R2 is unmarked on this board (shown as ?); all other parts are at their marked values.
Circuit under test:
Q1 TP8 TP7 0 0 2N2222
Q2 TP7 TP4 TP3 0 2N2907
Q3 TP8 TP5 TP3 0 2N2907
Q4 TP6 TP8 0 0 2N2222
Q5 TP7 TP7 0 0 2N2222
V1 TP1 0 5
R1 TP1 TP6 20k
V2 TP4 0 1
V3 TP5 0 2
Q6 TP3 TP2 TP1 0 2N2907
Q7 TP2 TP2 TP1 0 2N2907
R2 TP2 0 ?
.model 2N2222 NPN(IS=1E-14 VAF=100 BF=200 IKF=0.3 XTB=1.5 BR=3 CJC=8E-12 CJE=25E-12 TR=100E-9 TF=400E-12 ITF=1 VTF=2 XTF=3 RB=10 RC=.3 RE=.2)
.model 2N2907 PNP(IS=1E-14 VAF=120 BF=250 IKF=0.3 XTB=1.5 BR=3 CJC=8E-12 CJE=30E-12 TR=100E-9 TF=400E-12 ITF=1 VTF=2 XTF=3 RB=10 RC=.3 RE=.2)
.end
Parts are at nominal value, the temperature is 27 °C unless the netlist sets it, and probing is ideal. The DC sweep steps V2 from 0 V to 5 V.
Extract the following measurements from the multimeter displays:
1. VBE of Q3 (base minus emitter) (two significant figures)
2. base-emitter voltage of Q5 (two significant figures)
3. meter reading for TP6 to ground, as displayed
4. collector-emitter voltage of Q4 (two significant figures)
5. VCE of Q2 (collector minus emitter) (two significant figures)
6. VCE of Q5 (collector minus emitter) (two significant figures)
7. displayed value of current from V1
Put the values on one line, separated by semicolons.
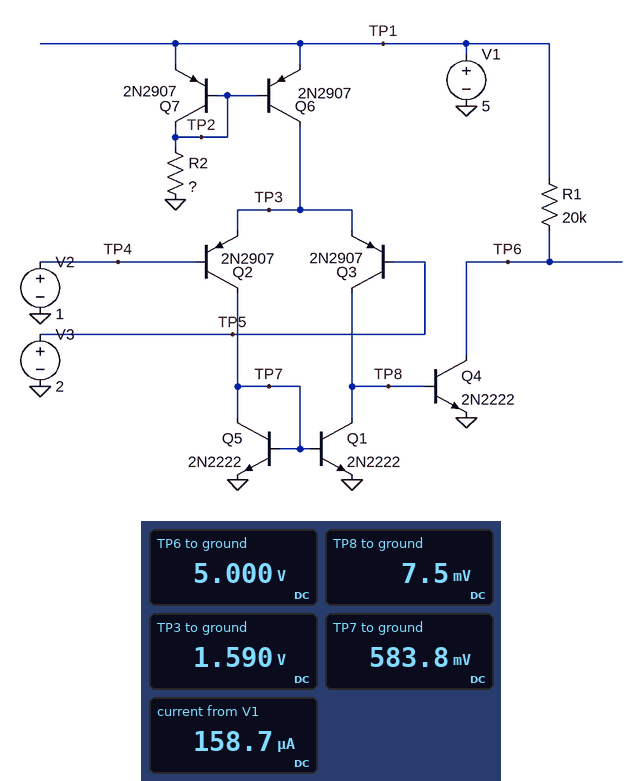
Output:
410 mV; 580 mV; 5.000 V; 5.0 V; -1.0 V; 580 mV; 158.7 µA
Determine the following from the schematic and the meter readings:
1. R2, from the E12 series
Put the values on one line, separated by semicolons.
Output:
56 kΩ
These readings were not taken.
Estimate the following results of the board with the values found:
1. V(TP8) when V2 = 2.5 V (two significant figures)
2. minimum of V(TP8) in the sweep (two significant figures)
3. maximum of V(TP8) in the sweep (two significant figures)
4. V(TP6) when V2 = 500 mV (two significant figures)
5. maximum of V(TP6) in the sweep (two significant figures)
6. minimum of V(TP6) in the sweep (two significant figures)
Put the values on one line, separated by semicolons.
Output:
640 mV; 7.5 mV; 640 mV; 5.0 V; 5.0 V; 23 mV
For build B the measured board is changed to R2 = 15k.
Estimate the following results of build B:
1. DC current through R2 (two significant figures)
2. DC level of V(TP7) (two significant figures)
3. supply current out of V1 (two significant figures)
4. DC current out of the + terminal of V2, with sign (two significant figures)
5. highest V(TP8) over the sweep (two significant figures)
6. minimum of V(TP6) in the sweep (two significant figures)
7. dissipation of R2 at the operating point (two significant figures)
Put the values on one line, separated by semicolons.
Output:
290 µA; 620 mV; 590 µA; -1.2 µA; 670 mV; 13 mV; 1.3 mW
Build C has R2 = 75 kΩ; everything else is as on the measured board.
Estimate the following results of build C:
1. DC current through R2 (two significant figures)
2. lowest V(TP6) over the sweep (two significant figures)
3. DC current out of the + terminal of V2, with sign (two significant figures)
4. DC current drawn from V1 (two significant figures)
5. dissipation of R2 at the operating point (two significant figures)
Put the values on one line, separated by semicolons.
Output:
59 µA; 27 mV; -240 nA; 120 µA; 260 µW
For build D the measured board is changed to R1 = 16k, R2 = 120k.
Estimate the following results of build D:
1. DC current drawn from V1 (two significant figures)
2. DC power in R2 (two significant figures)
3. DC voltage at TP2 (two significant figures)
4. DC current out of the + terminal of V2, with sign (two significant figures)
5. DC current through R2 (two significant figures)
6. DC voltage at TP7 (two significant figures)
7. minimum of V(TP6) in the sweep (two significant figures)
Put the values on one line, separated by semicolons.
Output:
74 µA; 160 µW; 4.4 V; -150 nA; 37 µA; 560 mV; 38 mV
